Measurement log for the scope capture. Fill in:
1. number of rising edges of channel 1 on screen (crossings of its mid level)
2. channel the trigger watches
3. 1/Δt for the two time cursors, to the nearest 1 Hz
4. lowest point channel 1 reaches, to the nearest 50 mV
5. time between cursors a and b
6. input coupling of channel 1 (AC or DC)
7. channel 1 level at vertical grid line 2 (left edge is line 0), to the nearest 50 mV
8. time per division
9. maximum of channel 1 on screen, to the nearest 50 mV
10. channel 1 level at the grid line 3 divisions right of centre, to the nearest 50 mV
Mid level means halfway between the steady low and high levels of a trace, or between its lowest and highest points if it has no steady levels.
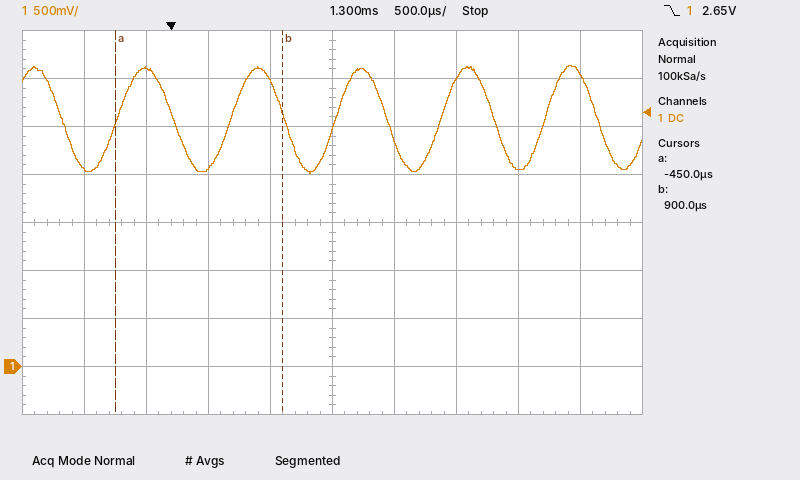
5
channel 1
741 Hz
2.00 V
1.35 ms
DC
3.10 V
500 µs
3.15 V
2.05 V
